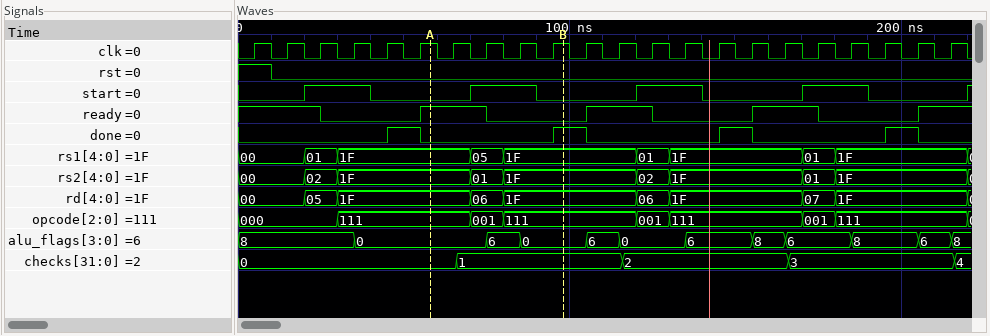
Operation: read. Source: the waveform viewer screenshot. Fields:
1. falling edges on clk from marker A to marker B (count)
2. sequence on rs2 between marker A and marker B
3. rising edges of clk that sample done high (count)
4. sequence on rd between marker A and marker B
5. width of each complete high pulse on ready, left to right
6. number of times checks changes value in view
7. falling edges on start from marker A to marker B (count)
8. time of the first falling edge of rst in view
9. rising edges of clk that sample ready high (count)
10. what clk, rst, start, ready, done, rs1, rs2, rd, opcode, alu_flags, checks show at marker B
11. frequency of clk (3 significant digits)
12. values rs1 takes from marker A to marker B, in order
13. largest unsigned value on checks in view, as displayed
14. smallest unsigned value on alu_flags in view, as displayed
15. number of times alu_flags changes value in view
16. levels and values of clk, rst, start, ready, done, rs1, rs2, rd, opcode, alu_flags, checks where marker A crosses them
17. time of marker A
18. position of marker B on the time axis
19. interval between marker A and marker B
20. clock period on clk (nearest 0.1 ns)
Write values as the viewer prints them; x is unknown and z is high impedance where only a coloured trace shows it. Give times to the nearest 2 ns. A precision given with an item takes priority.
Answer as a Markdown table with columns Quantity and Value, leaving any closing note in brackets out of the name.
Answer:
| Quantity | Value |
|---|---|
| falling edges on clk from marker A to marker B | 4 |
| sequence on rs2 between marker A and marker B | 1F, 01, 1F |
| rising edges of clk that sample done high | 4 |
| sequence on rd between marker A and marker B | 1F, 06, 1F |
| width of each complete high pulse on ready, left to right | 20 ns, 20 ns, 20 ns |
| number of times checks changes value in view | 4 |
| falling edges on start from marker A to marker B | 1 |
| time of the first falling edge of rst in view | 10 ns |
| rising edges of clk that sample ready high | 10 |
| what clk, rst, start, ready, done, rs1, rs2, rd, opcode, alu_flags, checks show at marker B | clk=1, rst=0, start=0, ready=0, done=1, rs1=1F, rs2=1F, rd=1F, opcode=111, alu_flags=0, checks=1 |
| frequency of clk | 100 MHz |
| values rs1 takes from marker A to marker B, in order | 1F, 05, 1F |
| largest unsigned value on checks in view, as displayed | 4 |
| smallest unsigned value on alu_flags in view, as displayed | 0 |
| number of times alu_flags changes value in view | 11 |
| levels and values of clk, rst, start, ready, done, rs1, rs2, rd, opcode, alu_flags, checks where marker A crosses them | clk=1, rst=0, start=0, ready=1, done=0, rs1=1F, rs2=1F, rd=1F, opcode=111, alu_flags=0, checks=0 |
| time of marker A | 58 ns |
| position of marker B on the time axis | 98 ns |
| interval between marker A and marker B | 40 ns |
| clock period on clk | 10 ns |
